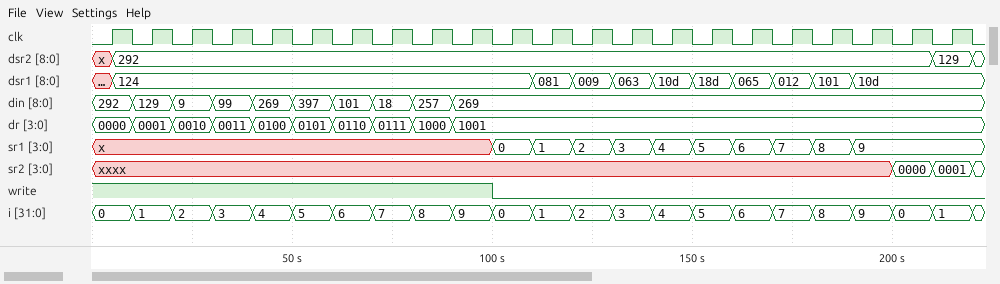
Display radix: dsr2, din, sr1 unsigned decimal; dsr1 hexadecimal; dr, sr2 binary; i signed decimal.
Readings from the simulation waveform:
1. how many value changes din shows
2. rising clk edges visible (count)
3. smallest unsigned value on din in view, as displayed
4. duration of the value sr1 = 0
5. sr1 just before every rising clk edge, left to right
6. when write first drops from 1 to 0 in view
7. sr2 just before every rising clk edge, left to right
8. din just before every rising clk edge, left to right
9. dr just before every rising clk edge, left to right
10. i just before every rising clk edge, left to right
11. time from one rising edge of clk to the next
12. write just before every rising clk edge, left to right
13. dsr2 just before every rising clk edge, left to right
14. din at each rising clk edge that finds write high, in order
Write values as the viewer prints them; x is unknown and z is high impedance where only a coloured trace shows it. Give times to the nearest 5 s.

9
22
9
10 s
x, x, x, x, x, x, x, x, x, x, 0, 1, 2, 3, 4, 5, 6, 7, 8, 9, 9, 9
100 s
xxxx, xxxx, xxxx, xxxx, xxxx, xxxx, xxxx, xxxx, xxxx, xxxx, xxxx, xxxx, xxxx, xxxx, xxxx, xxxx, xxxx, xxxx, xxxx, xxxx, 0000, 0001
292, 129, 9, 99, 269, 397, 101, 18, 257, 269, 269, 269, 269, 269, 269, 269, 269, 269, 269, 269, 269, 269
0000, 0001, 0010, 0011, 0100, 0101, 0110, 0111, 1000, 1001, 1001, 1001, 1001, 1001, 1001, 1001, 1001, 1001, 1001, 1001, 1001, 1001
0, 1, 2, 3, 4, 5, 6, 7, 8, 9, 0, 1, 2, 3, 4, 5, 6, 7, 8, 9, 0, 1
10 s
1 1 1 1 1 1 1 1 1 1 0 0 0 0 0 0 0 0 0 0 0 0
x, 292, 292, 292, 292, 292, 292, 292, 292, 292, 292, 292, 292, 292, 292, 292, 292, 292, 292, 292, 292, 129
292, 129, 9, 99, 269, 397, 101, 18, 257, 269
